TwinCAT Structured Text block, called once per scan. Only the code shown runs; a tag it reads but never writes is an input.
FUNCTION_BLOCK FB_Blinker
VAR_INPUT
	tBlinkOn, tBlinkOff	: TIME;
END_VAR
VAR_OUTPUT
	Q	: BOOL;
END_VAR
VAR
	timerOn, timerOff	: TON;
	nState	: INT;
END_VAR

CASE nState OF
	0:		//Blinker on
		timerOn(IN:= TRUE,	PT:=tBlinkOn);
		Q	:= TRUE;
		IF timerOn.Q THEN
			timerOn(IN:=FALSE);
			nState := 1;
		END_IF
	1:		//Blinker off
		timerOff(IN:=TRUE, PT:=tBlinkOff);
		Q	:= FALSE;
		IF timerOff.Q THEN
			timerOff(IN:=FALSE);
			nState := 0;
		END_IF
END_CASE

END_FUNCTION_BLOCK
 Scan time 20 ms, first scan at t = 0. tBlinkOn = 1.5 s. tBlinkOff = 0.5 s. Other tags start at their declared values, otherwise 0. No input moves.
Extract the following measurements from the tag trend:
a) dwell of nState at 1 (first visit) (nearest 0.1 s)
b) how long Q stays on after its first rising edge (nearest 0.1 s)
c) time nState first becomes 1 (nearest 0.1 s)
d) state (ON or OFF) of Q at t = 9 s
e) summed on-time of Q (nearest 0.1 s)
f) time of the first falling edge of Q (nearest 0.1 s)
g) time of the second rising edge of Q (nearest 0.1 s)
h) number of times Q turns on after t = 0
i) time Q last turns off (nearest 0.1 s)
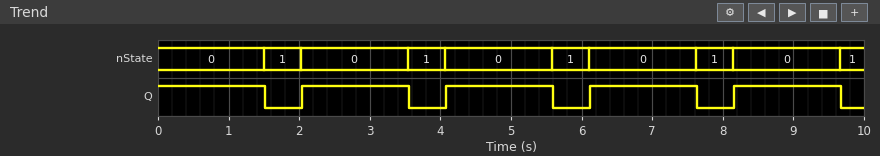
0.5 s
1.5 s
1.5 s
ON
7.6 s
1.5 s
4.1 s
4
9.7 s
